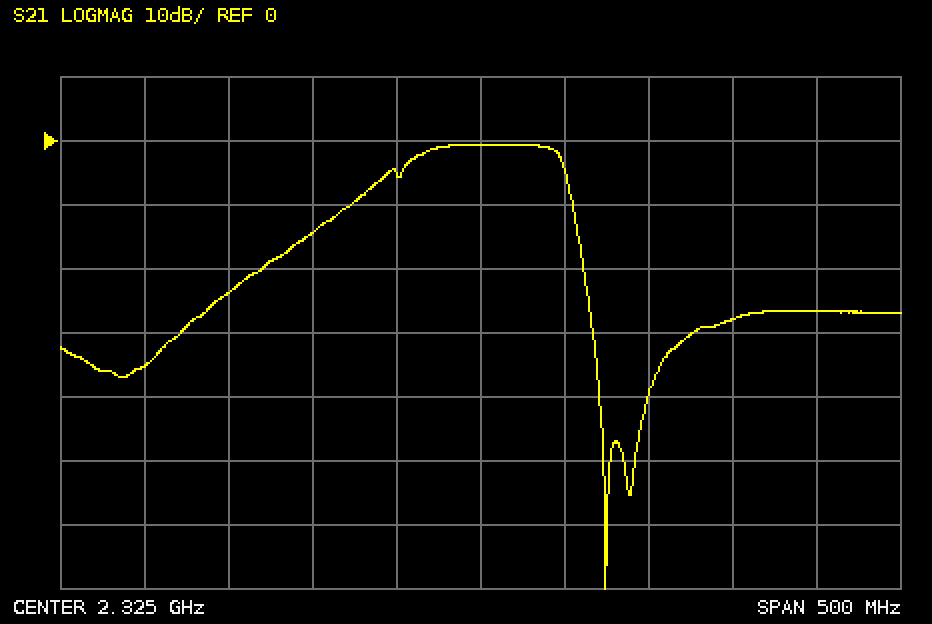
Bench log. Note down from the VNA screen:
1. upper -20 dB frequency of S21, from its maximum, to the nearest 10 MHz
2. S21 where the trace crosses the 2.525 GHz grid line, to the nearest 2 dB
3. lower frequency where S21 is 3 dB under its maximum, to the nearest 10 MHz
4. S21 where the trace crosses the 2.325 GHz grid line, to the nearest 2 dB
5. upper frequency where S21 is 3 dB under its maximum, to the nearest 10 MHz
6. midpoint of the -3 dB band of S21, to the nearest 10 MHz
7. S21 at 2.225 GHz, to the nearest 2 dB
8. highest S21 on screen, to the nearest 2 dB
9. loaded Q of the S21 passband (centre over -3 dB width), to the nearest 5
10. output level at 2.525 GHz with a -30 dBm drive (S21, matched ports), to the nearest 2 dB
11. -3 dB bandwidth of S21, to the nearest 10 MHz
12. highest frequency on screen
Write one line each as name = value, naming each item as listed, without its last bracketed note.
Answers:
upper -20 dB frequency of S21, from its maximum, to the nearest 10 MHz = 2.39 GHz
S21 where the trace crosses the 2.525 GHz grid line, to the nearest 2 dB = -26 dB
lower frequency where S21 is 3 dB under its maximum, to the nearest 10 MHz = 2.28 GHz
S21 where the trace crosses the 2.325 GHz grid line, to the nearest 2 dB = 0 dB
upper frequency where S21 is 3 dB under its maximum, to the nearest 10 MHz = 2.37 GHz
midpoint of the -3 dB band of S21, to the nearest 10 MHz = 2.33 GHz
S21 at 2.225 GHz, to the nearest 2 dB = -14 dB
highest S21 on screen, to the nearest 2 dB = 0 dB
loaded Q of the S21 passband (centre over -3 dB width), to the nearest 5 = 25
output level at 2.525 GHz with a -30 dBm drive (S21, matched ports), to the nearest 2 dB = -56 dBm
-3 dB bandwidth of S21, to the nearest 10 MHz = 90 MHz
highest frequency on screen = 2.575 GHz
